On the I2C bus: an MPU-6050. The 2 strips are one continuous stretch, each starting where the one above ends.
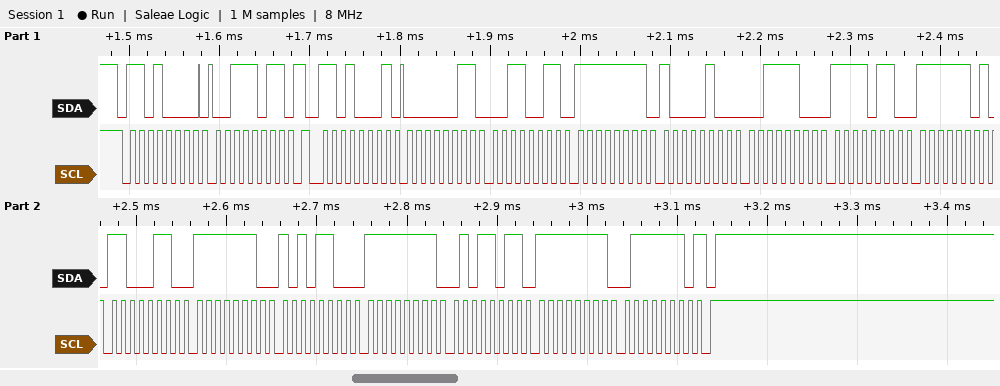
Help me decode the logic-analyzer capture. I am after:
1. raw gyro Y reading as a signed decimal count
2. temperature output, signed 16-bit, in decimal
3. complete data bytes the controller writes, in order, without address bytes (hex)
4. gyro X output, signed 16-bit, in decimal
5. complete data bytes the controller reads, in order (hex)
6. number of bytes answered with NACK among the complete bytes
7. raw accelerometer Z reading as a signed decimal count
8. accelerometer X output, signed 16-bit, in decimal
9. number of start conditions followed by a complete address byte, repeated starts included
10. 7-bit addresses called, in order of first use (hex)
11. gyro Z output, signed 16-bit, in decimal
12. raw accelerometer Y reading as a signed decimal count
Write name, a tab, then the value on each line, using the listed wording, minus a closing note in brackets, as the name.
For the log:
raw gyro Y reading as a signed decimal count	-165
temperature output, signed 16-bit, in decimal	-570
complete data bytes the controller writes, in order, without address bytes	3B
gyro X output, signed 16-bit, in decimal	-340
complete data bytes the controller reads, in order	03 33 FF 84 3C F6 FD C6 FE AC FF 5B FF 7E
number of bytes answered with NACK among the complete bytes	1
raw accelerometer Z reading as a signed decimal count	15606
accelerometer X output, signed 16-bit, in decimal	819
number of start conditions followed by a complete address byte, repeated starts included	2
7-bit addresses called, in order of first use	0x68
gyro Z output, signed 16-bit, in decimal	-130
raw accelerometer Y reading as a signed decimal count	-124
